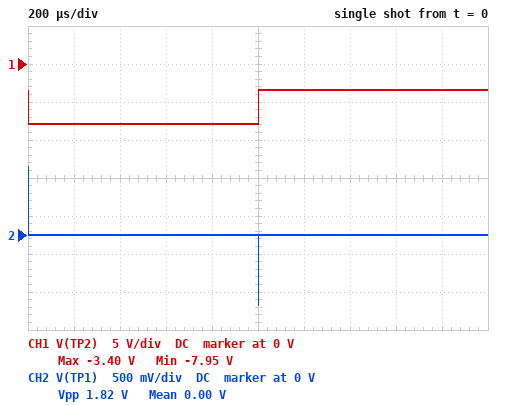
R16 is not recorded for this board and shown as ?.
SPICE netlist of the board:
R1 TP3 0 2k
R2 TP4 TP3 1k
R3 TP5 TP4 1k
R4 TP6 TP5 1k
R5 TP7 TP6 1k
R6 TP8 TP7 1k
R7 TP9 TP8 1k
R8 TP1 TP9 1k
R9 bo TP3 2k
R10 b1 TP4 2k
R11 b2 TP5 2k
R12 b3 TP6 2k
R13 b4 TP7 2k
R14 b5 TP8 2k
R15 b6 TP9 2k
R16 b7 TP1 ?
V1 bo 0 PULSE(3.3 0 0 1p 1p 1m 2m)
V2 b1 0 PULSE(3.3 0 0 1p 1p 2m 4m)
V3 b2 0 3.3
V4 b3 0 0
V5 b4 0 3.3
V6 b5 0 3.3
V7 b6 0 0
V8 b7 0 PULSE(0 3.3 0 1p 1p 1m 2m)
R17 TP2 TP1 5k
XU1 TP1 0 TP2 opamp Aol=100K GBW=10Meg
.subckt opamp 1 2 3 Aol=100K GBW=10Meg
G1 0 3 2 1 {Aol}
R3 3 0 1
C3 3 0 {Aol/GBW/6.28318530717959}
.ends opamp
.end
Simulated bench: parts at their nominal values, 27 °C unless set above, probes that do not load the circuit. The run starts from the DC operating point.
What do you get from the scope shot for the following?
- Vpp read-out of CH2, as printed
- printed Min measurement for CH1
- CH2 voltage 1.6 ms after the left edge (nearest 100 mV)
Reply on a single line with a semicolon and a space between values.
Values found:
1.82 V; -7.95 V; 0 V
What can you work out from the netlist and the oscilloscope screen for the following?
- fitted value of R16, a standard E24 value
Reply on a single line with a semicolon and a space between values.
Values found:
3.6 kΩ
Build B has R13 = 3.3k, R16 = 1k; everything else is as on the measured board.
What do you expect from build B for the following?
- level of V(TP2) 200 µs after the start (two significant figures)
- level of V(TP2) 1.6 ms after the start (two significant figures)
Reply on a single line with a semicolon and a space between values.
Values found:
-20 V; -3.2 V
